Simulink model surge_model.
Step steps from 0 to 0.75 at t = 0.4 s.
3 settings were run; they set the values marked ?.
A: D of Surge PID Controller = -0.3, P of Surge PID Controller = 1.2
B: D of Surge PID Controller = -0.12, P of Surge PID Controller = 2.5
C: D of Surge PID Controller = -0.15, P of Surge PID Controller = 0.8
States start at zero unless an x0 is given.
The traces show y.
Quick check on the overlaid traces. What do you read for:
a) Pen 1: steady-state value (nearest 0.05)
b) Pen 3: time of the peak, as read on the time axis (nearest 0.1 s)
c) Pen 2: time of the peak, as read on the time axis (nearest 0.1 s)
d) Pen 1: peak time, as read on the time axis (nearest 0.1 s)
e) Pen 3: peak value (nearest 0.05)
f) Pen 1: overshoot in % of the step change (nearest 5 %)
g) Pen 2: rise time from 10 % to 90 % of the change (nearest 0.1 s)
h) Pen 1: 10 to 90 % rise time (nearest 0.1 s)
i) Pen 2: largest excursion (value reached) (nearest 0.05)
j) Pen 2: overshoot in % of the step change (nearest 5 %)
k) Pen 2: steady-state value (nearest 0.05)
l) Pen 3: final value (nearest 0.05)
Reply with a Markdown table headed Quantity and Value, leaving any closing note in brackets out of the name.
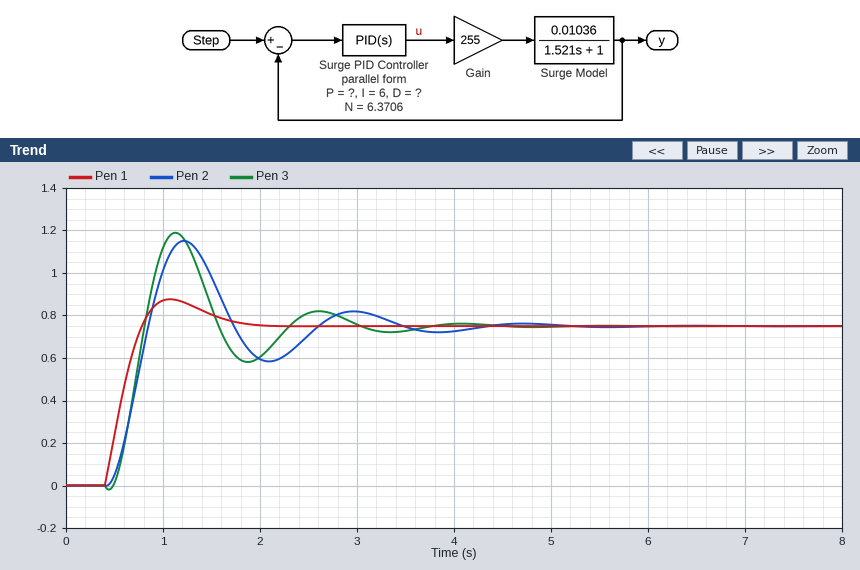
| Quantity | Value |
|---|---|
| Pen 1: steady-state value | 0.75 |
| Pen 3: time of the peak, as read on the time axis | 1.1 s |
| Pen 2: time of the peak, as read on the time axis | 1.2 s |
| Pen 1: peak time, as read on the time axis | 1.1 s |
| Pen 3: peak value | 1.20 |
| Pen 1: overshoot in % of the step change | 15 % |
| Pen 2: rise time from 10 % to 90 % of the change | 0.3 s |
| Pen 1: 10 to 90 % rise time | 0.3 s |
| Pen 2: largest excursion (value reached) | 1.15 |
| Pen 2: overshoot in % of the step change | 55 % |
| Pen 2: steady-state value | 0.75 |
| Pen 3: final value | 0.75 |
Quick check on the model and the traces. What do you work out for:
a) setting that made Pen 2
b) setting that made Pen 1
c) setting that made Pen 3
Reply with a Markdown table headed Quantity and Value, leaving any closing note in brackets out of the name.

| Quantity | Value |
|---|---|
| setting that made Pen 2 | C |
| setting that made Pen 1 | B |
| setting that made Pen 3 | A |
